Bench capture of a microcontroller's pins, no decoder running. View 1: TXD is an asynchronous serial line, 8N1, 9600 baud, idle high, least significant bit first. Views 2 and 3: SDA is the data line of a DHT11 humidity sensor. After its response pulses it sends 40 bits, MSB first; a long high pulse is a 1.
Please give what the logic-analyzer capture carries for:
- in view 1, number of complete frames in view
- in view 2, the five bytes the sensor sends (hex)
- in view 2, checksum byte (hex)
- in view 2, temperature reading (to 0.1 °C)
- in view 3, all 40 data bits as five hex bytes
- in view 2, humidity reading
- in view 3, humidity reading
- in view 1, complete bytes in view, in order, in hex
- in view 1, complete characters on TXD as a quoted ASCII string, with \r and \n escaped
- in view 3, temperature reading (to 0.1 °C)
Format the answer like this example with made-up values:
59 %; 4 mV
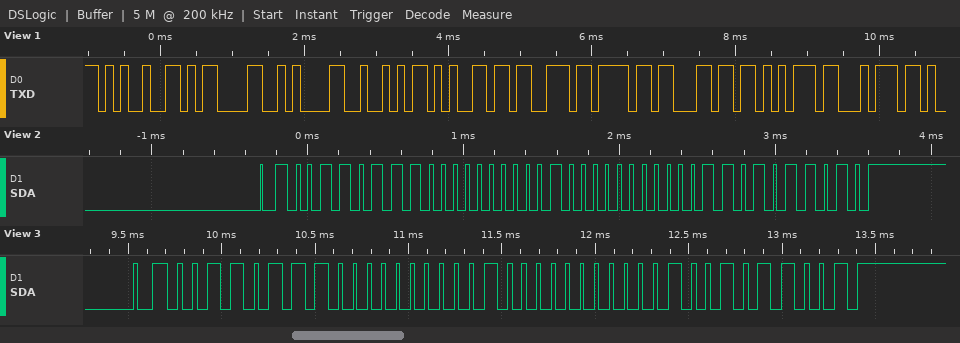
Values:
10; 37 00 20 03 5A; 0x5A; 32.3 °C; 37 00 20 02 59; 55 %; 55 %; 25 0D 0A 52 65 73 6F 6C 75 74; "%\r\nResolut"; 32.2 °C
